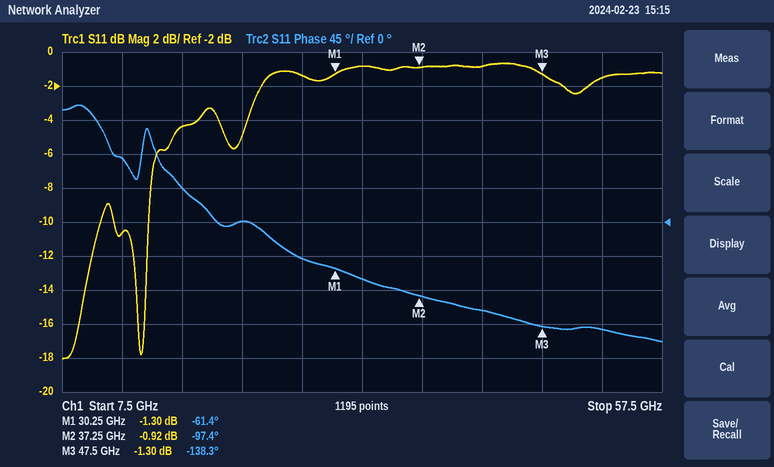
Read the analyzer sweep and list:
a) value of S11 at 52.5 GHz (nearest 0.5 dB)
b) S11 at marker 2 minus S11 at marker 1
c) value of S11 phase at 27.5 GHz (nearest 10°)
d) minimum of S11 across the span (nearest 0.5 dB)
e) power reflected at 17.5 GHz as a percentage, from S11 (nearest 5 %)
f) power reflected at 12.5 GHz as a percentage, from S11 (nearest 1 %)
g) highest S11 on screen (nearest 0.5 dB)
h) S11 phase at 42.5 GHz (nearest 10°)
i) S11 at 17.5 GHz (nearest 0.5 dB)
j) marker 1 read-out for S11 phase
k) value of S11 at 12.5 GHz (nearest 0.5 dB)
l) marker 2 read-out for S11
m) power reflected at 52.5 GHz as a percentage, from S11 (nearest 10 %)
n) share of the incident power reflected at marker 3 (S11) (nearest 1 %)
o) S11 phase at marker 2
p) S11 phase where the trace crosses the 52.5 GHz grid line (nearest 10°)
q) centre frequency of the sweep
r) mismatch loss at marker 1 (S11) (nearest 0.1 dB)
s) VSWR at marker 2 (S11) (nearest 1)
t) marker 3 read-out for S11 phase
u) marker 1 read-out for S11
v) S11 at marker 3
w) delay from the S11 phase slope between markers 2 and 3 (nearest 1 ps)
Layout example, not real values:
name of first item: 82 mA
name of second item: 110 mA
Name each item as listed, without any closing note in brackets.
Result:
value of S11 at 52.5 GHz: -1.5 dB
S11 at marker 2 minus S11 at marker 1: 0.38 dB
value of S11 phase at 27.5 GHz: -50°
minimum of S11 across the span: -18.0 dB
power reflected at 17.5 GHz as a percentage, from S11: 35 %
power reflected at 12.5 GHz as a percentage, from S11: 9 %
highest S11 on screen: -0.5 dB
S11 phase at 42.5 GHz: -120°
S11 at 17.5 GHz: -4.5 dB
marker 1 read-out for S11 phase: -61.4°
value of S11 at 12.5 GHz: -10.5 dB
marker 2 read-out for S11: -0.92 dB
power reflected at 52.5 GHz as a percentage, from S11: 70 %
share of the incident power reflected at marker 3 (S11): 74 %
S11 phase at marker 2: -97.4°
S11 phase where the trace crosses the 52.5 GHz grid line: -140°
centre frequency of the sweep: 32.5 GHz
mismatch loss at marker 1 (S11): 5.9 dB
VSWR at marker 2 (S11): 19
marker 3 read-out for S11 phase: -138.3°
marker 1 read-out for S11: -1.30 dB
S11 at marker 3: -1.30 dB
delay from the S11 phase slope between markers 2 and 3: 11 ps
